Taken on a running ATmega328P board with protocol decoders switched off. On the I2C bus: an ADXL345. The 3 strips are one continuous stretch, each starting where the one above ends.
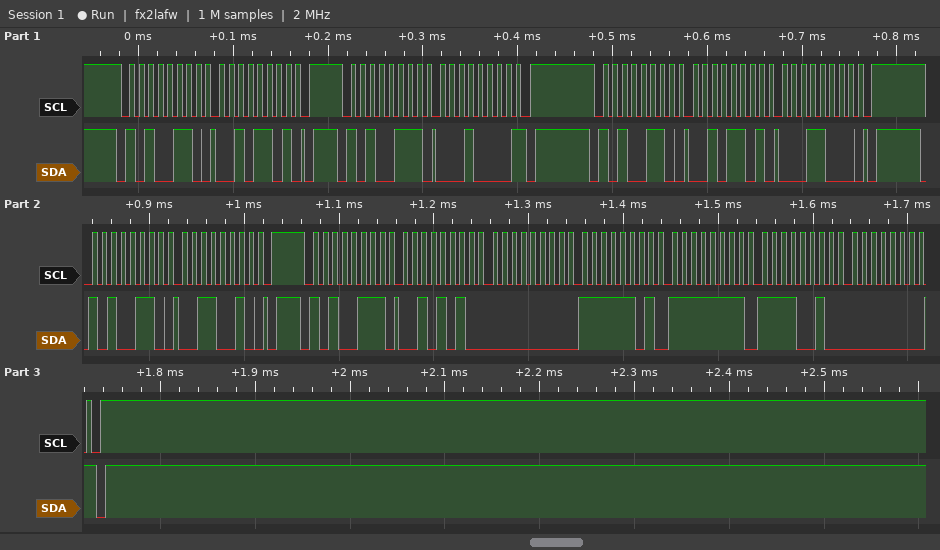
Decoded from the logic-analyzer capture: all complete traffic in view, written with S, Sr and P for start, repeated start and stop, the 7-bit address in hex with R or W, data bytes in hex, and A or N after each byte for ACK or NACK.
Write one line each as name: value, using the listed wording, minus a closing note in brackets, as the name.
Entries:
all complete traffic in view, written with S, Sr and P for start, repeated start and stop, the 7-bit address in hex with R or W, data bytes in hex, and A or N after each byte for ACK or NACK: S 53W A 2D A P S 53R A 10 N P S 53W A 2D A 18 A P S 53W A 32 A P S 53R A 2A A 00 A FD A FF A F2 A 00 N P
